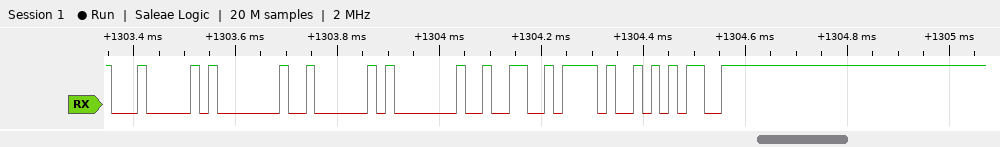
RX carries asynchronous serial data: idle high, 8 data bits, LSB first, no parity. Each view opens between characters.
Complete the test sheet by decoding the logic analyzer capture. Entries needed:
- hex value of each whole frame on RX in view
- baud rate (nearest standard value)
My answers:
04, 01, 02, 01, 32, 2F, 35
57600 baud
